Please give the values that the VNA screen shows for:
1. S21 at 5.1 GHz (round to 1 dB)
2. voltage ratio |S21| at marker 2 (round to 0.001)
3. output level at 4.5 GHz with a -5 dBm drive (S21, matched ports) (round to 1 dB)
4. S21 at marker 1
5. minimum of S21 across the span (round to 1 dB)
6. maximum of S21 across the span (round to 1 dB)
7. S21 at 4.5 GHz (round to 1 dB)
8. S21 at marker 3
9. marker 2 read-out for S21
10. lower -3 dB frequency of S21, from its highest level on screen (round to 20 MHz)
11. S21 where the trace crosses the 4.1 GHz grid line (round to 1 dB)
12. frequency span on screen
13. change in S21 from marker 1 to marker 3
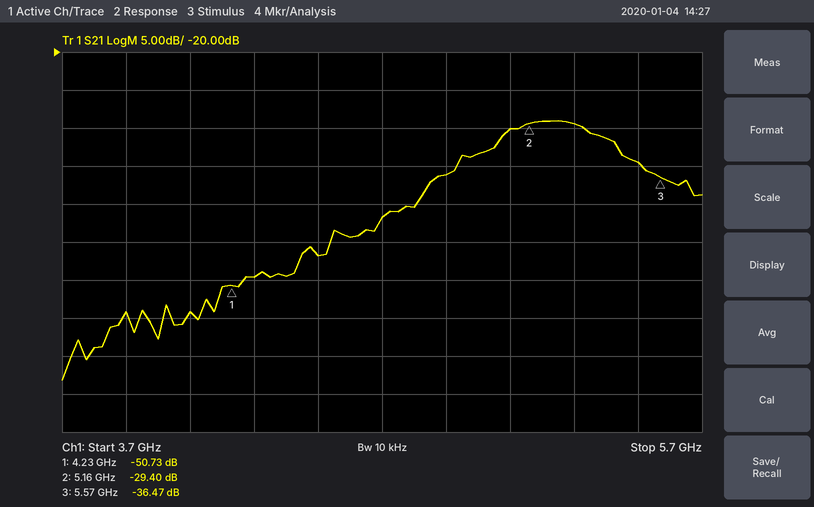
-30 dB
0.034
-52 dBm
-50.73 dB
-63 dB
-29 dB
-47 dB
-36.47 dB
-29.40 dB
5.06 GHz
-54 dB
2 GHz
14.26 dB
